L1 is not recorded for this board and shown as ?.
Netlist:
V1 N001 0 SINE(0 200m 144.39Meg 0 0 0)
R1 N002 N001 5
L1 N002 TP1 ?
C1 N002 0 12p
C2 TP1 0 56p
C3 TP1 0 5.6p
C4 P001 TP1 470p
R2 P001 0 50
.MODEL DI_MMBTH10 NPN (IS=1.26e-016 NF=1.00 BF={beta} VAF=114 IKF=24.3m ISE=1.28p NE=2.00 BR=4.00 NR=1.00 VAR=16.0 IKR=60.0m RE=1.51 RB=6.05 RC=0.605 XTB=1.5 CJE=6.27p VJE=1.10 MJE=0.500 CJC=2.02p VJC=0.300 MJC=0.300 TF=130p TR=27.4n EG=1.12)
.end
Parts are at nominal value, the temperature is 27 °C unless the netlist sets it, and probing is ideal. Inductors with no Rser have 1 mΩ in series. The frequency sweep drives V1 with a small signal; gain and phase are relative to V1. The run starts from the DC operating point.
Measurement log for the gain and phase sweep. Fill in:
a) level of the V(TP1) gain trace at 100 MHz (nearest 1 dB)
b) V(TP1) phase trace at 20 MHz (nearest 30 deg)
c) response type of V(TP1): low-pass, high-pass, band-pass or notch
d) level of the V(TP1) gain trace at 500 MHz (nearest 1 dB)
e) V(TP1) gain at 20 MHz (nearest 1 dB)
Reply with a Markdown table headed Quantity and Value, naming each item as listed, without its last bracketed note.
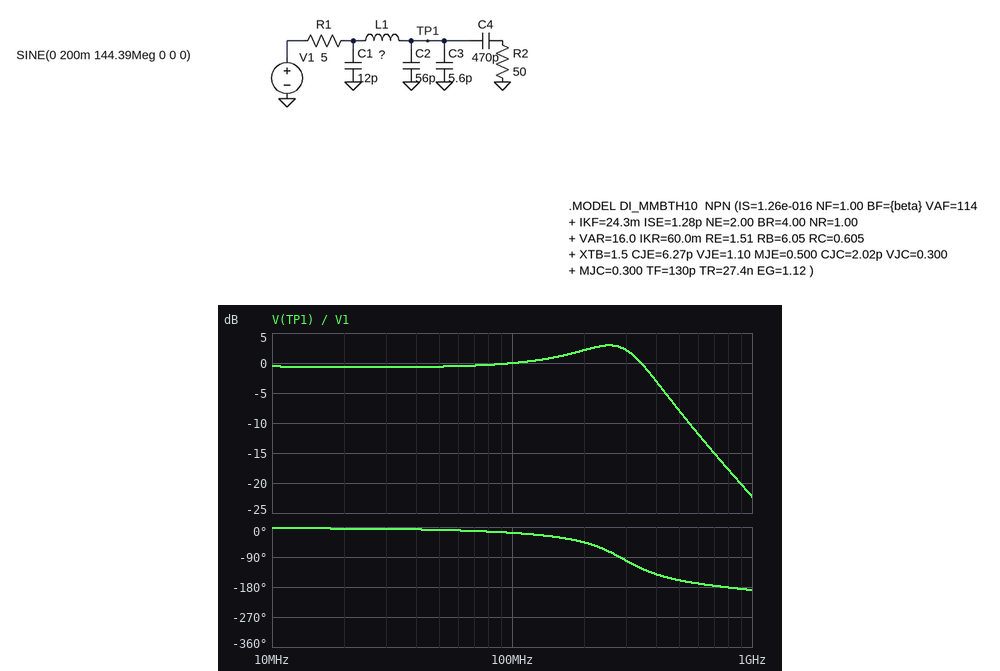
| Quantity | Value |
|---|---|
| level of the V(TP1) gain trace at 100 MHz | 0 dB |
| V(TP1) phase trace at 20 MHz | 0 deg |
| response type of V(TP1): low-pass, high-pass, band-pass or notch | low-pass |
| level of the V(TP1) gain trace at 500 MHz | -8 dB |
| V(TP1) gain at 20 MHz | -1 dB |
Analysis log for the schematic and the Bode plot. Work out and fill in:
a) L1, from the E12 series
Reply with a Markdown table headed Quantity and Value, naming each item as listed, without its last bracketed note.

| Quantity | Value |
|---|---|
| L1, from the E12 series | 5.6 nH |
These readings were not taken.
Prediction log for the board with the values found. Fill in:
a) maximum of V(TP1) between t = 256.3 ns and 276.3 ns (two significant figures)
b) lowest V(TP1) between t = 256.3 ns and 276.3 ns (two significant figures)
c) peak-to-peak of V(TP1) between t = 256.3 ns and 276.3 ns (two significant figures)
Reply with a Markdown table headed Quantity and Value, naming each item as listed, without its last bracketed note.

| Quantity | Value |
|---|---|
| maximum of V(TP1) between t = 256.3 ns and 276.3 ns | 220 mV |
| lowest V(TP1) between t = 256.3 ns and 276.3 ns | -220 mV |
| peak-to-peak of V(TP1) between t = 256.3 ns and 276.3 ns | 440 mV |
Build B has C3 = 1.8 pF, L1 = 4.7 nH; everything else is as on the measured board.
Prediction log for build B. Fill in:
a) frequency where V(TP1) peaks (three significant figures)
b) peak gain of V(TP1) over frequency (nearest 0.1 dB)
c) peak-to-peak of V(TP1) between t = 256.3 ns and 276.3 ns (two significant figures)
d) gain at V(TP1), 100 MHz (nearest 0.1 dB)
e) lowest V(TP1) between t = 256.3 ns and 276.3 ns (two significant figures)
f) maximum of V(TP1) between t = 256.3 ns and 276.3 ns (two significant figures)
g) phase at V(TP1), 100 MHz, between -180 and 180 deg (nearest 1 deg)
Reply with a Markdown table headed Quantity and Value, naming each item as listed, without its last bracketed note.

| Quantity | Value |
|---|---|
| frequency where V(TP1) peaks | 286 MHz |
| peak gain of V(TP1) over frequency | 2.7 dB |
| peak-to-peak of V(TP1) between t = 256.3 ns and 276.3 ns | 420 mV |
| gain at V(TP1), 100 MHz | -0.2 dB |
| lowest V(TP1) between t = 256.3 ns and 276.3 ns | -210 mV |
| maximum of V(TP1) between t = 256.3 ns and 276.3 ns | 210 mV |
| phase at V(TP1), 100 MHz, between -180 and 180 deg | -16 deg |
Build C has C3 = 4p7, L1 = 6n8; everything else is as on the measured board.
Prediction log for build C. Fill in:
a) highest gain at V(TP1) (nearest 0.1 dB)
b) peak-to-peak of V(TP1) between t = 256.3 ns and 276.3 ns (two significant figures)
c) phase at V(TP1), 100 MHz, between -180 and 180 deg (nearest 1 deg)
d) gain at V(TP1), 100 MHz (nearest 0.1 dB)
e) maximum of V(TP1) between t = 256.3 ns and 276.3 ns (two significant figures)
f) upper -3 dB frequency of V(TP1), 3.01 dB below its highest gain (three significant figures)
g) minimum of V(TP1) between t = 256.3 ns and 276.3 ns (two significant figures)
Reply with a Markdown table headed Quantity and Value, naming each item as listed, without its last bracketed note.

| Quantity | Value |
|---|---|
| highest gain at V(TP1) | 3.3 dB |
| peak-to-peak of V(TP1) between t = 256.3 ns and 276.3 ns | 460 mV |
| phase at V(TP1), 100 MHz, between -180 and 180 deg | -19 deg |
| gain at V(TP1), 100 MHz | 0.2 dB |
| maximum of V(TP1) between t = 256.3 ns and 276.3 ns | 230 mV |
| upper -3 dB frequency of V(TP1), 3.01 dB below its highest gain | 314 MHz |
| minimum of V(TP1) between t = 256.3 ns and 276.3 ns | -230 mV |
